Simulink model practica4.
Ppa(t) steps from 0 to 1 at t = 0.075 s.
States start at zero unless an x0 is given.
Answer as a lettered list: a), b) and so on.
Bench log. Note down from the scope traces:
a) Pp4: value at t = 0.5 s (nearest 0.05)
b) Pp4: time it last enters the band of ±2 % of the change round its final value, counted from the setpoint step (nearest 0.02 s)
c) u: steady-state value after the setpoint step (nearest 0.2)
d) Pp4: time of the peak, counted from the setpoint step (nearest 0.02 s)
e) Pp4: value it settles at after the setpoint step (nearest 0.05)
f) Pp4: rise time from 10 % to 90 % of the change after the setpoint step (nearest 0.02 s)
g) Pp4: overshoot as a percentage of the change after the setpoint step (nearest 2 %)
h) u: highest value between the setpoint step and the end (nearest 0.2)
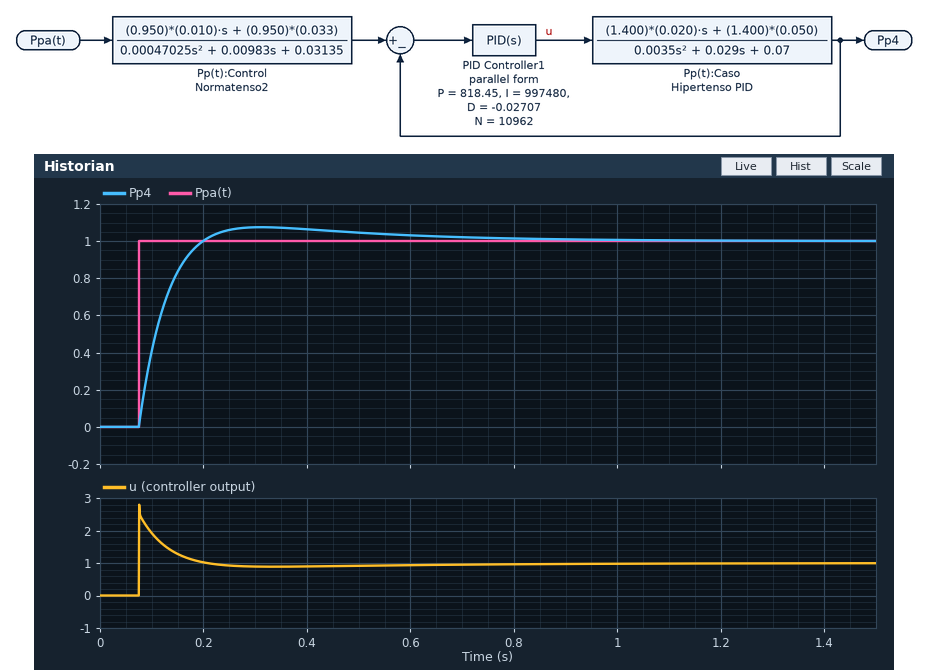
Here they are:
a) 1.05
b) 0.64 s
c) 1.0
d) 0.24 s
e) 1.00
f) 0.08 s
g) 8 %
h) 2.8
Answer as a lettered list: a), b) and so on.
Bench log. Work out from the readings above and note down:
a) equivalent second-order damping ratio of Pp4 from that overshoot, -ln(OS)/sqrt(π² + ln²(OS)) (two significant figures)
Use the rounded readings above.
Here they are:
a) 0.63
